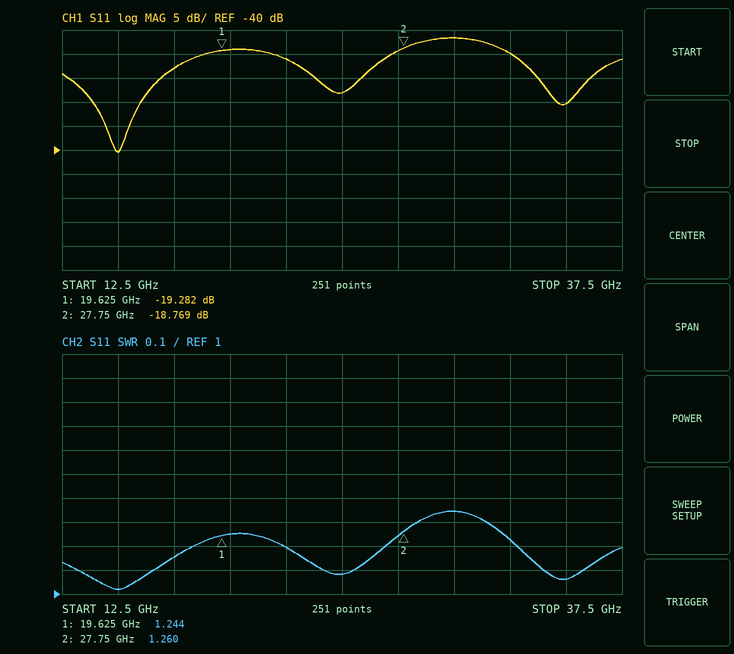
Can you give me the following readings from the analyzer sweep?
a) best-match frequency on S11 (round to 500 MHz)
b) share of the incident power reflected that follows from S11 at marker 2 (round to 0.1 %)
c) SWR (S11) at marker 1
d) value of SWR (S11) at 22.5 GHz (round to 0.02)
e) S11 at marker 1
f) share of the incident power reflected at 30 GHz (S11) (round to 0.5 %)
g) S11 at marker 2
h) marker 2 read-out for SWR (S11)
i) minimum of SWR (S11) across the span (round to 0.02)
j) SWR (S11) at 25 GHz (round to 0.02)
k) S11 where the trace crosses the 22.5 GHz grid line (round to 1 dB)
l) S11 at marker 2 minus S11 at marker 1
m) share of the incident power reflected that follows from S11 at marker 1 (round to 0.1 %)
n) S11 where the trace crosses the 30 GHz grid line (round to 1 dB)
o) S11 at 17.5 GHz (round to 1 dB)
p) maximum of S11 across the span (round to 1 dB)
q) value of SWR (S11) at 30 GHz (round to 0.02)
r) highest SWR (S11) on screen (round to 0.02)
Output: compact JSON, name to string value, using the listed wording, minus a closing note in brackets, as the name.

{"best-match frequency on S11": "15.0 GHz", "share of the incident power reflected that follows from S11 at marker 2": "1.3 %", "SWR (S11) at marker 1": "1.244", "value of SWR (S11) at 22.5 GHz": "1.20", "S11 at marker 1": "-19.282 dB", "share of the incident power reflected at 30 GHz (S11)": "2.0 %", "S11 at marker 2": "-18.769 dB", "marker 2 read-out for SWR": "1.260", "minimum of SWR (S11) across the span": "1.02", "SWR (S11) at 25 GHz": "1.08", "S11 where the trace crosses the 22.5 GHz grid line": "-21 dB", "S11 at marker 2 minus S11 at marker 1": "0.513 dB", "share of the incident power reflected that follows from S11 at marker 1": "1.2 %", "S11 where the trace crosses the 30 GHz grid line": "-17 dB", "S11 at 17.5 GHz": "-23 dB", "maximum of S11 across the span": "-17 dB", "value of SWR (S11) at 30 GHz": "1.34", "highest SWR (S11) on screen": "1.34"}
